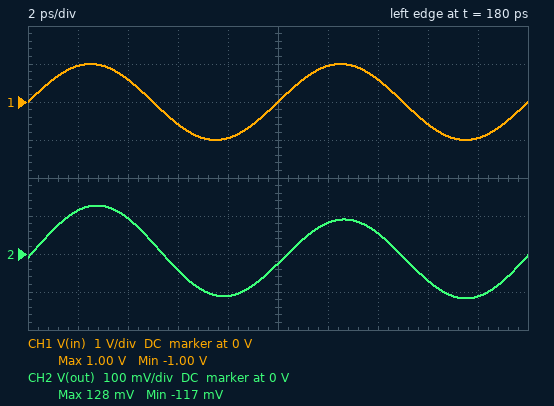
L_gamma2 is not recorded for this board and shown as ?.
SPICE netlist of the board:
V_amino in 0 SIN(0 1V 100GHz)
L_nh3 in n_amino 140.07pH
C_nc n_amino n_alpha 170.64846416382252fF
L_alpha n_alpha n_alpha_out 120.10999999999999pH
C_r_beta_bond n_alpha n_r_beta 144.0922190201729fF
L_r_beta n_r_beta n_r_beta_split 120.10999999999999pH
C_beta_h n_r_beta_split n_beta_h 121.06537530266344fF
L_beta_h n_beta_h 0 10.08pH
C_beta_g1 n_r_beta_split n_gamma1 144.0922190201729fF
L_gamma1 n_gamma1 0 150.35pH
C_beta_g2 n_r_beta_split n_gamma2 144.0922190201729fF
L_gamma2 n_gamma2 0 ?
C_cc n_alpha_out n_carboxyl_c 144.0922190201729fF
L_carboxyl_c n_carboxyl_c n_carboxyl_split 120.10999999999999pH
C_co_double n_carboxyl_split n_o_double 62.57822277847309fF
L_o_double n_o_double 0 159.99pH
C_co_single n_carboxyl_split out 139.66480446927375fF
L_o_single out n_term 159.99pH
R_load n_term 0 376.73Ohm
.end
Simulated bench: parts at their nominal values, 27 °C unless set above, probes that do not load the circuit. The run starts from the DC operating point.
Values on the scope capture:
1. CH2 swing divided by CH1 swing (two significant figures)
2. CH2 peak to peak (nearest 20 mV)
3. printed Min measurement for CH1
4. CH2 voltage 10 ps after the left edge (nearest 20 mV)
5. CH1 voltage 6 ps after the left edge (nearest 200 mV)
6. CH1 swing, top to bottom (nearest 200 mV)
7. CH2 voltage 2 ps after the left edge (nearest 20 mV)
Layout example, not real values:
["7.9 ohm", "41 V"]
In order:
["0.12", "240 mV", "-1.00 V", "-20 mV", "-600 mV", "2.0 V", "120 mV"]
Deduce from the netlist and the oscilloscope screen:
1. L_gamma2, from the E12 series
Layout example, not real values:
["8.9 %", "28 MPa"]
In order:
["56 pH"]
